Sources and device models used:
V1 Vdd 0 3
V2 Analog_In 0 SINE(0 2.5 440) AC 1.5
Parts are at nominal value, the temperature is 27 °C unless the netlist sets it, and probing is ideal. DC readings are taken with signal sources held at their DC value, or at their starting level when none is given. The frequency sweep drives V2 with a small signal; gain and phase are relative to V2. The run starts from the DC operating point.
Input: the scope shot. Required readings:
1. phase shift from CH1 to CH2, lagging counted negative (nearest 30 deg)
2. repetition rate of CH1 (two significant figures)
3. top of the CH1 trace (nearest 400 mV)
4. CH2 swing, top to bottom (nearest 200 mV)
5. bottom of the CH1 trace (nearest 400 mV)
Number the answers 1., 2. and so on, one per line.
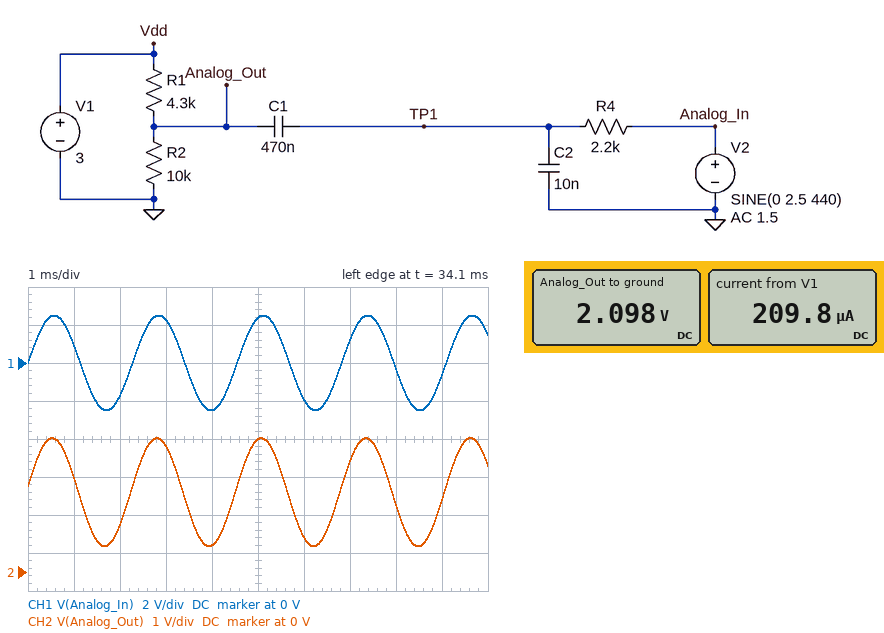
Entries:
1. 0 deg
2. 440 Hz
3. 2.4 V
4. 2.8 V
5. -2.4 V
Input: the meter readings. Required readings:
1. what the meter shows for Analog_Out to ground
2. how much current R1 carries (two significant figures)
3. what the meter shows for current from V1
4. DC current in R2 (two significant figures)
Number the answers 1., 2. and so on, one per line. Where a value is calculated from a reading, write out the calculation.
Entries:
1. 2.098 V
2. (3 V - 2.098 V) / 4.3 kΩ = 210 µA
3. 209.8 µA
4. (2.098 V) / 10 kΩ = 210 µA
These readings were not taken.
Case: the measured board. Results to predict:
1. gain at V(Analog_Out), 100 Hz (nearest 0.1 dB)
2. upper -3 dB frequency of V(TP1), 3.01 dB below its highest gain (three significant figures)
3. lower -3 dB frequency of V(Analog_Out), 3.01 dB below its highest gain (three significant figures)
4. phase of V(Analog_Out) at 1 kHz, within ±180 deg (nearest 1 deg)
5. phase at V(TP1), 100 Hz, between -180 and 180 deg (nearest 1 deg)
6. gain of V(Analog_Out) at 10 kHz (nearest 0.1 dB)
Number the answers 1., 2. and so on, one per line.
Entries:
1. -6.3 dB
2. 111 Hz
3. 64.1 Hz
4. -1 deg
5. -16 deg
6. -6.9 dB
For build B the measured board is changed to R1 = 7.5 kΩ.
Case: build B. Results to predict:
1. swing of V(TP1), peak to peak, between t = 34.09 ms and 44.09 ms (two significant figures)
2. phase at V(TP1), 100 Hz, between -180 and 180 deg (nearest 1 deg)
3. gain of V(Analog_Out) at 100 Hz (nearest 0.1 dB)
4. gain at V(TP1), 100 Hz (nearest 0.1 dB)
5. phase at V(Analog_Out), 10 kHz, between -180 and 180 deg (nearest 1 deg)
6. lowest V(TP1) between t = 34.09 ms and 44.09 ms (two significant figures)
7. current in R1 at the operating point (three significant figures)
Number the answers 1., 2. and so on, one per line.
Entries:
1. 3.3 V
2. -11 deg
3. -4.7 dB
4. -2.6 dB
5. -42 deg
6. -1.7 V
7. 171 µA
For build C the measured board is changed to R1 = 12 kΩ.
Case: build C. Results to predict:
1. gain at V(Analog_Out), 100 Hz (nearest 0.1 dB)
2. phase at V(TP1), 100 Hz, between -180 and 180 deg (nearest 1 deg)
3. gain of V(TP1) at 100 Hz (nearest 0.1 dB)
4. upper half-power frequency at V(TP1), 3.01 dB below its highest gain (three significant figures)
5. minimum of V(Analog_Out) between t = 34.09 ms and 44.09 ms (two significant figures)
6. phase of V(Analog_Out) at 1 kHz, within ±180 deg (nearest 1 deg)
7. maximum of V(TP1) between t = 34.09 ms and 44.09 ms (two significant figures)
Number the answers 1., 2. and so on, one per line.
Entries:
1. -3.7 dB
2. -9 deg
3. -2.3 dB
4. 1.18 kHz
5. -400 mV
6. -3 deg
7. 1.8 V
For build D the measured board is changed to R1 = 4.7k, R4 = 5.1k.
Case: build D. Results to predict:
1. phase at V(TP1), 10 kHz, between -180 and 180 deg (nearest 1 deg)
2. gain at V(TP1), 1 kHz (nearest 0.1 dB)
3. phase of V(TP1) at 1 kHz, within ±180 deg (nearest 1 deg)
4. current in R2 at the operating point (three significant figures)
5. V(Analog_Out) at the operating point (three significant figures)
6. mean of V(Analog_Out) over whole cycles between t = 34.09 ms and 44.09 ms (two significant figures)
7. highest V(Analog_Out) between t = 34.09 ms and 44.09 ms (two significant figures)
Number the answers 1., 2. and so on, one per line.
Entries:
1. -51 deg
2. -8.4 dB
3. -11 deg
4. 204 µA
5. 2.04 V
6. 2.0 V
7. 3.0 V
